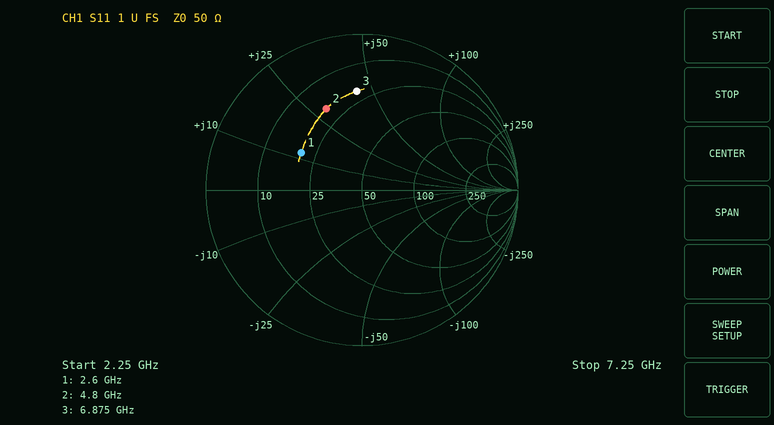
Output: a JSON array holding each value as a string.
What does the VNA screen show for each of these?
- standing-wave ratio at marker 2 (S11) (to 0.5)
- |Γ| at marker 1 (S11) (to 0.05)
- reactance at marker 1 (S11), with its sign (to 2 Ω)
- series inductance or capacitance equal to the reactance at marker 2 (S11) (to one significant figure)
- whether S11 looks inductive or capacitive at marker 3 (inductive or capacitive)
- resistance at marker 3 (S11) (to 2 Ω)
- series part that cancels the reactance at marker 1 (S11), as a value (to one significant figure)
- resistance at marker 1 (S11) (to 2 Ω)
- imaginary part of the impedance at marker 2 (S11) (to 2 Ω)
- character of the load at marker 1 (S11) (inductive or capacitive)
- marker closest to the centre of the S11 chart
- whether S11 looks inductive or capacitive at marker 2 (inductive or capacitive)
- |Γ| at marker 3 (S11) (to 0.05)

["3.5", "0.45", "+12 Ω", "1.0 nH", "inductive", "20 Ω", "5 pF", "20 Ω", "+30 Ω", "inductive", "marker 1", "inductive", "0.65"]
